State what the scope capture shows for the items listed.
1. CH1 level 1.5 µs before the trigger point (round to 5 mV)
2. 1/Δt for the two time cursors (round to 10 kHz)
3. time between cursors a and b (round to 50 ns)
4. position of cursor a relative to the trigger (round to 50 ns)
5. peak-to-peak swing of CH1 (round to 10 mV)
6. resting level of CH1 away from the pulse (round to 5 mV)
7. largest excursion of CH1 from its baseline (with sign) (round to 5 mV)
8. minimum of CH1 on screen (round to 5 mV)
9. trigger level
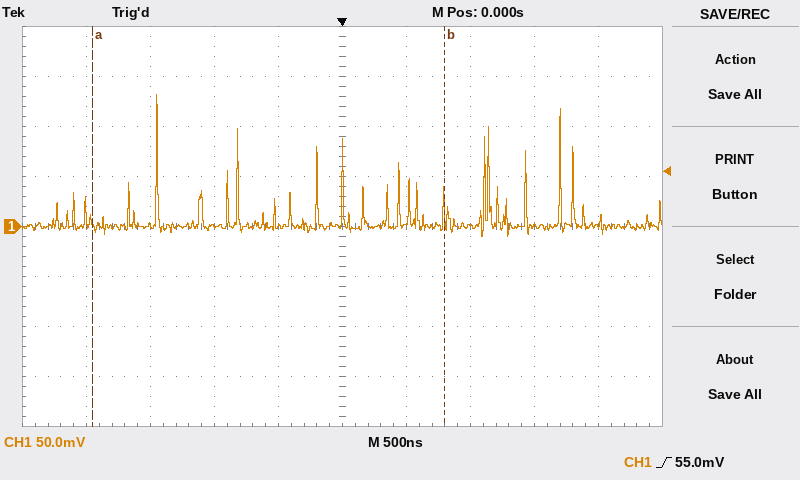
0 mV
360 kHz
2.75 µs
-1.95 µs
140 mV
0 mV
+130 mV
-10 mV
55.0 mV
